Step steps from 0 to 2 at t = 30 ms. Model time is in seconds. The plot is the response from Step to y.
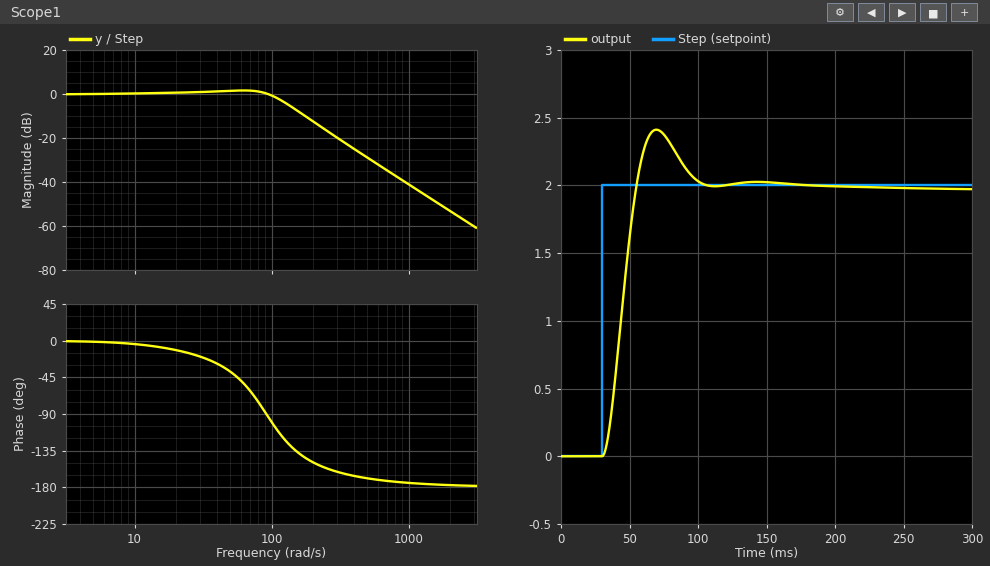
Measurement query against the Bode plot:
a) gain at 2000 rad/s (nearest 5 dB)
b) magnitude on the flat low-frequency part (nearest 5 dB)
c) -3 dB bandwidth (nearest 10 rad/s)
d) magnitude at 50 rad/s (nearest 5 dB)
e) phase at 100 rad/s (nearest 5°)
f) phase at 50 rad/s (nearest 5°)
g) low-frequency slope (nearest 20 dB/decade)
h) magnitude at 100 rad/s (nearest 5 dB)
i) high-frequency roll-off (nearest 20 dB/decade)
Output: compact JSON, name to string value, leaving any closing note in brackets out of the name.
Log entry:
{"gain at 2000 rad/s": "-55 dB", "magnitude on the flat low-frequency part": "0 dB", "-3 dB bandwidth": "120 rad/s", "magnitude at 50 rad/s": "0 dB", "phase at 100 rad/s": "-100°", "phase at 50 rad/s": "-40°", "low-frequency slope": "0 dB/decade", "magnitude at 100 rad/s": "0 dB", "high-frequency roll-off": "-40 dB/decade"}
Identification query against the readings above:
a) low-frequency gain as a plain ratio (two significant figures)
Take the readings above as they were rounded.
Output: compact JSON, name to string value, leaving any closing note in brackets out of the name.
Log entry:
{"low-frequency gain as a plain ratio": "1.0"}
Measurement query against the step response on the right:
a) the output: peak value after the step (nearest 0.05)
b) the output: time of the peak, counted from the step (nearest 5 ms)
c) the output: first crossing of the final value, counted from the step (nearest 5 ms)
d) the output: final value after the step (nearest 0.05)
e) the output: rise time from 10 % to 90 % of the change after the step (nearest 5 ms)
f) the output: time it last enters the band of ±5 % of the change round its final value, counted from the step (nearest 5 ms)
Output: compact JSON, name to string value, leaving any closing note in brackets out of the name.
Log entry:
{"the output: peak value after the step": "2.40", "the output: time of the peak, counted from the step": "40 ms", "the output: first crossing of the final value, counted from the step": "25 ms", "the output: final value after the step": "1.95", "the output: rise time from 10 % to 90 % of the change after the step": "15 ms", "the output: time it last enters the band of ±5 % of the change round its final value, counted from the step": "65 ms"}
